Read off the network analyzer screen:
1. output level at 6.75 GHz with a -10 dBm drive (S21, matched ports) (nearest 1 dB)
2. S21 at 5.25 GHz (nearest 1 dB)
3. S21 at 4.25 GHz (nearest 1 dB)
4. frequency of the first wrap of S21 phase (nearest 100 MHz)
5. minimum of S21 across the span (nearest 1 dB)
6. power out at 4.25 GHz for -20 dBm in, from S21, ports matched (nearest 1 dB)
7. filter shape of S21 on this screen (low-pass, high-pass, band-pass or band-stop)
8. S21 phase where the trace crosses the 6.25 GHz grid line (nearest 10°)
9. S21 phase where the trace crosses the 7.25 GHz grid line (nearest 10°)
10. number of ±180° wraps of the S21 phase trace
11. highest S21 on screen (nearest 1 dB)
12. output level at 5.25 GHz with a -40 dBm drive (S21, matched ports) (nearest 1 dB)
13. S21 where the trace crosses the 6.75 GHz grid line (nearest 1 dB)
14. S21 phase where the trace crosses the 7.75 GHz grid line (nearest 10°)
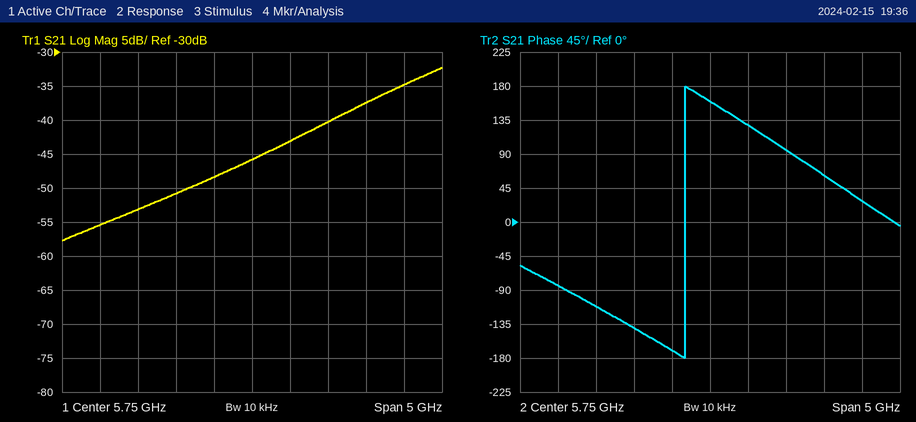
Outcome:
-50 dBm
-48 dB
-53 dB
5.4 GHz
-58 dB
-73 dBm
high-pass
130°
60°
1
-32 dB
-88 dBm
-40 dB
30°
